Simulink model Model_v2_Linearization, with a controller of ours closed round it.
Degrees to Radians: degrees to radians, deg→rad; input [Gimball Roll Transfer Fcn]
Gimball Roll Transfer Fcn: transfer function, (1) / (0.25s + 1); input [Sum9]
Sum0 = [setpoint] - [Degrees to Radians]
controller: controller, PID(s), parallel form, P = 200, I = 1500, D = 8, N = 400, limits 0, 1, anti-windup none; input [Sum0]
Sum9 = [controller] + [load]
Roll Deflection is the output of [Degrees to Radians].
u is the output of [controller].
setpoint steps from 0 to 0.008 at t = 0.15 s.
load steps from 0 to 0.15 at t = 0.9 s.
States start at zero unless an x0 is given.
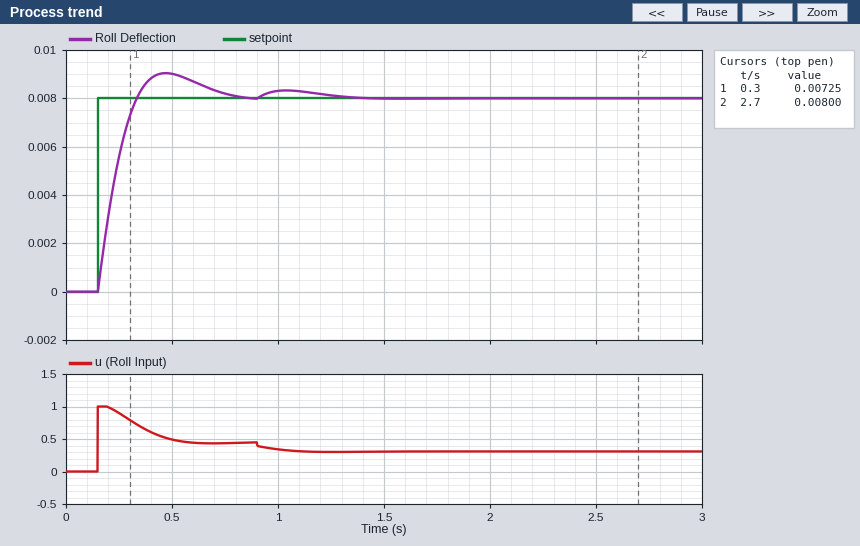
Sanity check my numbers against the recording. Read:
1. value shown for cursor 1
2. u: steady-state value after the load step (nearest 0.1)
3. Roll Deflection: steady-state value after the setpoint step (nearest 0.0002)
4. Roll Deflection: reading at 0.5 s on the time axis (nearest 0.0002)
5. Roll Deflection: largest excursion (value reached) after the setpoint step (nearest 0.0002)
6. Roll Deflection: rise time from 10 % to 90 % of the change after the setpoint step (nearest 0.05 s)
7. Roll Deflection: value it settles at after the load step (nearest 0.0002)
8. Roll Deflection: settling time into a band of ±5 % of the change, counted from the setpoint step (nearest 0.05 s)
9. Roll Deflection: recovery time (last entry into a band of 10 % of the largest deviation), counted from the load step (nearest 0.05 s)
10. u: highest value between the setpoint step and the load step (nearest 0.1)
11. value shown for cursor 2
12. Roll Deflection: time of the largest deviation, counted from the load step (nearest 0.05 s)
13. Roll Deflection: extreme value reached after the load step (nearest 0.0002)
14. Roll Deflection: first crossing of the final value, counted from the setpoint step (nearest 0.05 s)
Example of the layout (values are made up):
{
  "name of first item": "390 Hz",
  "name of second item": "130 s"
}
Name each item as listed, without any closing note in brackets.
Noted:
{
  "value shown for cursor 1": "0.00725",
  "u: steady-state value after the load step": "0.3",
  "Roll Deflection: steady-state value after the setpoint step": "0.0080",
  "Roll Deflection: reading at 0.5 s on the time axis": "0.0090",
  "Roll Deflection: largest excursion (value reached) after the setpoint step": "0.0090",
  "Roll Deflection: rise time from 10 % to 90 % of the change after the setpoint step": "0.15 s",
  "Roll Deflection: value it settles at after the load step": "0.0080",
  "Roll Deflection: settling time into a band of ±5 % of the change, counted from the setpoint step": "0.55 s",
  "Roll Deflection: recovery time (last entry into a band of 10 % of the largest deviation), counted from the load step": "0.45 s",
  "u: highest value between the setpoint step and the load step": "1.0",
  "value shown for cursor 2": "0.00800",
  "Roll Deflection: time of the largest deviation, counted from the load step": "0.15 s",
  "Roll Deflection: extreme value reached after the load step": "0.0084",
  "Roll Deflection: first crossing of the final value, counted from the setpoint step": "0.20 s"
}
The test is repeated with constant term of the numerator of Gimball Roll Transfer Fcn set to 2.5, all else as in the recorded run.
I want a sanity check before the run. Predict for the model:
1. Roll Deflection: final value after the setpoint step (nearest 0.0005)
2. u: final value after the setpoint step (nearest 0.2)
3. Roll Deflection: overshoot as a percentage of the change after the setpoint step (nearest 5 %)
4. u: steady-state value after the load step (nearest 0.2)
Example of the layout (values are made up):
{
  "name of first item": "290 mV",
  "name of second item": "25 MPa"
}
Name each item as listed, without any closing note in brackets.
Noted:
{
  "Roll Deflection: final value after the setpoint step": "0.0080",
  "u: final value after the setpoint step": "0.2",
  "Roll Deflection: overshoot as a percentage of the change after the setpoint step": "15 %",
  "u: steady-state value after the load step": "0.0"
}
